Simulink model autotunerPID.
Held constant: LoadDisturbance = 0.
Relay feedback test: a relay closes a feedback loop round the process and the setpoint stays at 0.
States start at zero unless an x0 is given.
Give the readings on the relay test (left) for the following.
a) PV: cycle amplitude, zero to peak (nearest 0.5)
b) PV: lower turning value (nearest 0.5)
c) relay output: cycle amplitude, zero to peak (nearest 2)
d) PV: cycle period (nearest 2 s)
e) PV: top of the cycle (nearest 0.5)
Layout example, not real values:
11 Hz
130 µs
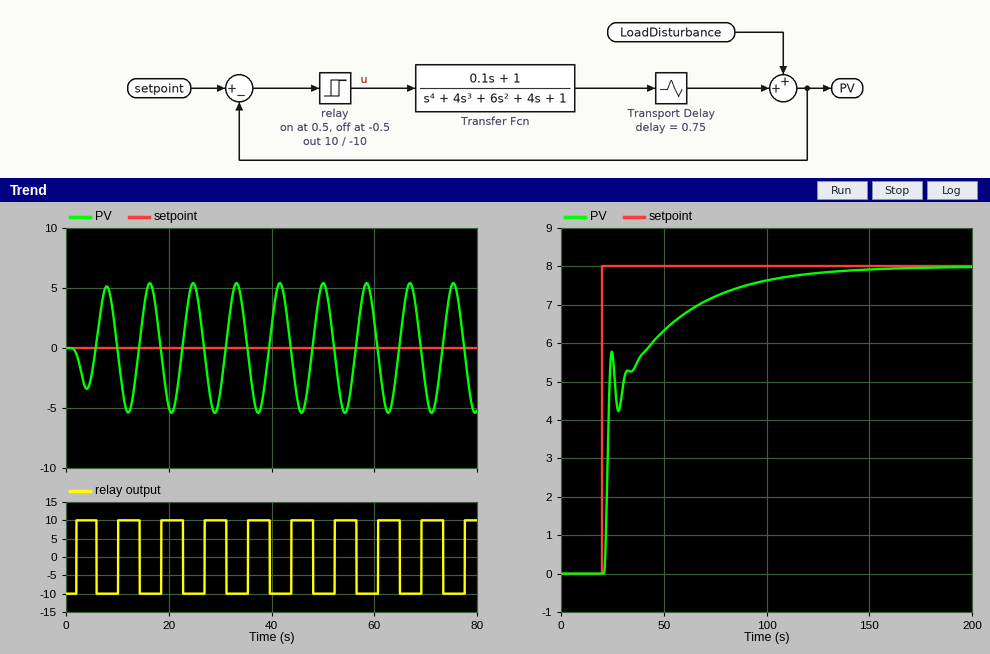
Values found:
5.5
-5.5
10
8 s
5.5
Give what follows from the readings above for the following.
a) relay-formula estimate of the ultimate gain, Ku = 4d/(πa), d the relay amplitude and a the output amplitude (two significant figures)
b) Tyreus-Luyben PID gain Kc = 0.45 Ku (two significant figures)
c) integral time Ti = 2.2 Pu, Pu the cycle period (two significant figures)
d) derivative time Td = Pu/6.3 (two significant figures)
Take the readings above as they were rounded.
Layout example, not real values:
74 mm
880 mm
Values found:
2.3
1.0
18 s
1.3 s
